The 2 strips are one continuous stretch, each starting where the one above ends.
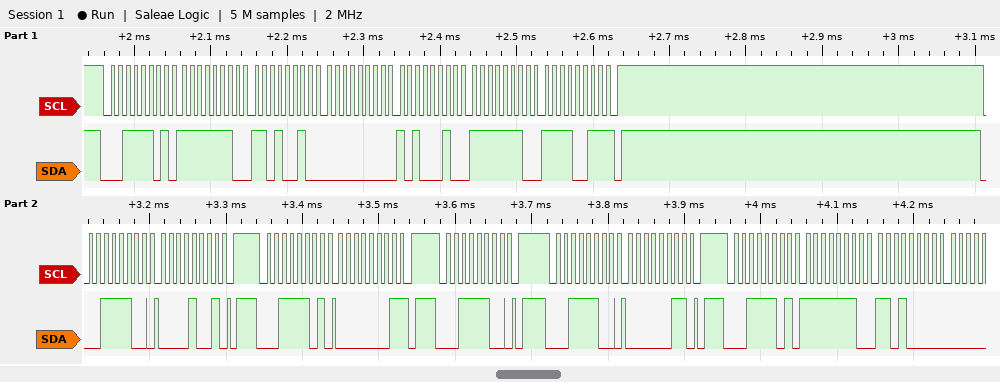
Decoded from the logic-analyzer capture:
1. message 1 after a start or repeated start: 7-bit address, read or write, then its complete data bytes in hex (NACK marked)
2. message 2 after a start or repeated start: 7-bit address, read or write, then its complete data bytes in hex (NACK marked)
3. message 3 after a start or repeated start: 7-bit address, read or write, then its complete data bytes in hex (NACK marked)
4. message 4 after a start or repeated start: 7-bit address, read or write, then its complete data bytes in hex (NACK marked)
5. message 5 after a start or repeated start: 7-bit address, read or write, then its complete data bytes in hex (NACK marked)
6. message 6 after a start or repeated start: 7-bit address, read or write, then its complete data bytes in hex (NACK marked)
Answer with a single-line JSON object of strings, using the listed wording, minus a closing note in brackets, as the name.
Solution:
{"message 1 after a start or repeated start: 7-bit address, read or write, then its complete data bytes in hex": "0x1E read: FE D2 00 A2 FE F3 NACK", "message 2 after a start or repeated start: 7-bit address, read or write, then its complete data bytes in hex": "0x1E write: 09", "message 3 after a start or repeated start: 7-bit address, read or write, then its complete data bytes in hex": "0x1E read: 01 NACK", "message 4 after a start or repeated start: 7-bit address, read or write, then its complete data bytes in hex": "0x1E write", "message 5 after a start or repeated start: 7-bit address, read or write, then its complete data bytes in hex": "0x1E write: 03", "message 6 after a start or repeated start: 7-bit address, read or write, then its complete data bytes in hex": "0x1E read: FE D0"}
